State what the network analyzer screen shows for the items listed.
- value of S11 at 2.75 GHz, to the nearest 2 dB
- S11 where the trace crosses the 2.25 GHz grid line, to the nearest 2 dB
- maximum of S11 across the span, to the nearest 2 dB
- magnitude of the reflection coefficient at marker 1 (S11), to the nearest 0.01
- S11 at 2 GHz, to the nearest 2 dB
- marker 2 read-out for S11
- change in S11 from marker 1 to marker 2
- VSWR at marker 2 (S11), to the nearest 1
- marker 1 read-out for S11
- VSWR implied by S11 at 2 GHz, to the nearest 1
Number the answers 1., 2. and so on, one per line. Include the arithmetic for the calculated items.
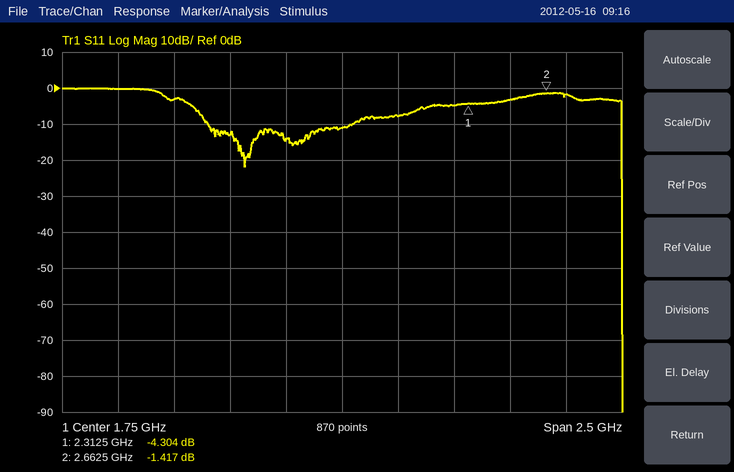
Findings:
1. -2 dB
2. -4 dB
3. 0 dB
4. 10^(-4.304/20) ≈ 0.61
5. -8 dB
6. -1.417 dB
7. -1.417 − (-4.304) = 2.887 dB
8. (1 + 0.8495)/(1 − 0.8495) ≈ 12
9. -4.304 dB
10. |Γ| = 10^(-8/20) = 0.3981; VSWR = (1 + 0.3981)/(1 − 0.3981) ≈ 2
